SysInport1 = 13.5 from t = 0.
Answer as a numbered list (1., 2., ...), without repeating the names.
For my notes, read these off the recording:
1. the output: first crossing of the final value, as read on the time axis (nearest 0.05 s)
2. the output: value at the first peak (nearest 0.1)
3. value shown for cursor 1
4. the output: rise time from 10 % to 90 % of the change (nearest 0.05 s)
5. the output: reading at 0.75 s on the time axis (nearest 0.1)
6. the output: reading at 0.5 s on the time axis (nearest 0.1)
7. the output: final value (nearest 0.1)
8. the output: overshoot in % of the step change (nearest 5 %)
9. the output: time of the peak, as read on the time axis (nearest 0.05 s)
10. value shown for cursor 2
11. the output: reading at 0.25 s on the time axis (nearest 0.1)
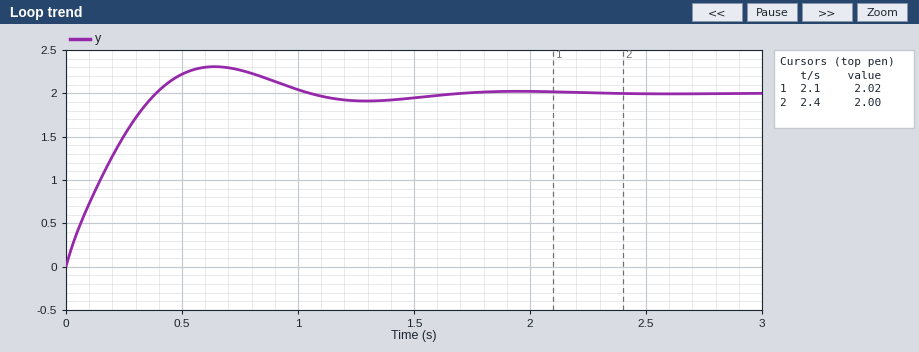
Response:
1. 0.40 s
2. 2.3
3. 2.02
4. 0.30 s
5. 2.3
6. 2.2
7. 2.0
8. 15 %
9. 0.65 s
10. 2.00
11. 1.5
